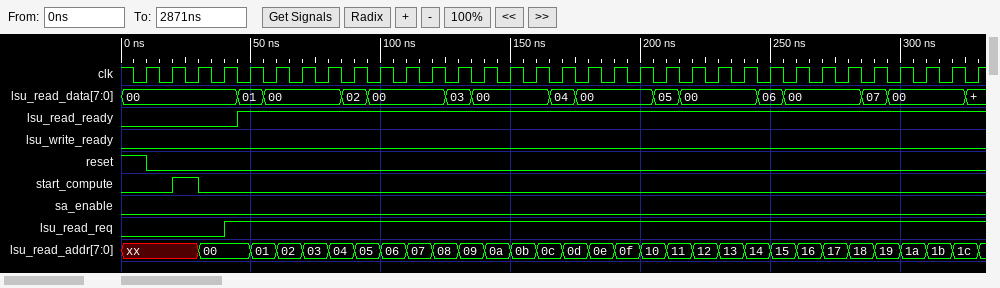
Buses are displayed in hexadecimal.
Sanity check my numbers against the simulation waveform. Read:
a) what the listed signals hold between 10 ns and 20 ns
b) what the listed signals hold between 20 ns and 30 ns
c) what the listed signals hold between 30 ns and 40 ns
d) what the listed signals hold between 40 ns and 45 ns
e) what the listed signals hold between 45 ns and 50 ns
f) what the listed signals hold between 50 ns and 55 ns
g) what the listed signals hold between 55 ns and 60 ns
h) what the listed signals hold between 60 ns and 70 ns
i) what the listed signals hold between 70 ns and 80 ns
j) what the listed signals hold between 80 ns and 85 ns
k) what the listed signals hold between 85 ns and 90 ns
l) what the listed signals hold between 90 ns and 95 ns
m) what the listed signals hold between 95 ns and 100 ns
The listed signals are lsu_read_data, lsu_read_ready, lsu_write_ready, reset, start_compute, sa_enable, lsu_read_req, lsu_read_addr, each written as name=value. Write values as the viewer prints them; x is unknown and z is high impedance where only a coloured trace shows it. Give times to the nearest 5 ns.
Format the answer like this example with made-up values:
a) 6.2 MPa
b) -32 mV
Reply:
a) lsu_read_data=00, lsu_read_ready=0, lsu_write_ready=0, reset=0, start_compute=0, sa_enable=0, lsu_read_req=0, lsu_read_addr=xx
b) lsu_read_data=00, lsu_read_ready=0, lsu_write_ready=0, reset=0, start_compute=1, sa_enable=0, lsu_read_req=0, lsu_read_addr=xx
c) lsu_read_data=00, lsu_read_ready=0, lsu_write_ready=0, reset=0, start_compute=0, sa_enable=0, lsu_read_req=0, lsu_read_addr=00
d) lsu_read_data=00, lsu_read_ready=0, lsu_write_ready=0, reset=0, start_compute=0, sa_enable=0, lsu_read_req=1, lsu_read_addr=00
e) lsu_read_data=01, lsu_read_ready=1, lsu_write_ready=0, reset=0, start_compute=0, sa_enable=0, lsu_read_req=1, lsu_read_addr=00
f) lsu_read_data=01, lsu_read_ready=1, lsu_write_ready=0, reset=0, start_compute=0, sa_enable=0, lsu_read_req=1, lsu_read_addr=01
g) lsu_read_data=00, lsu_read_ready=1, lsu_write_ready=0, reset=0, start_compute=0, sa_enable=0, lsu_read_req=1, lsu_read_addr=01
h) lsu_read_data=00, lsu_read_ready=1, lsu_write_ready=0, reset=0, start_compute=0, sa_enable=0, lsu_read_req=1, lsu_read_addr=02
i) lsu_read_data=00, lsu_read_ready=1, lsu_write_ready=0, reset=0, start_compute=0, sa_enable=0, lsu_read_req=1, lsu_read_addr=03
j) lsu_read_data=00, lsu_read_ready=1, lsu_write_ready=0, reset=0, start_compute=0, sa_enable=0, lsu_read_req=1, lsu_read_addr=04
k) lsu_read_data=02, lsu_read_ready=1, lsu_write_ready=0, reset=0, start_compute=0, sa_enable=0, lsu_read_req=1, lsu_read_addr=04
l) lsu_read_data=02, lsu_read_ready=1, lsu_write_ready=0, reset=0, start_compute=0, sa_enable=0, lsu_read_req=1, lsu_read_addr=05
m) lsu_read_data=00, lsu_read_ready=1, lsu_write_ready=0, reset=0, start_compute=0, sa_enable=0, lsu_read_req=1, lsu_read_addr=05
